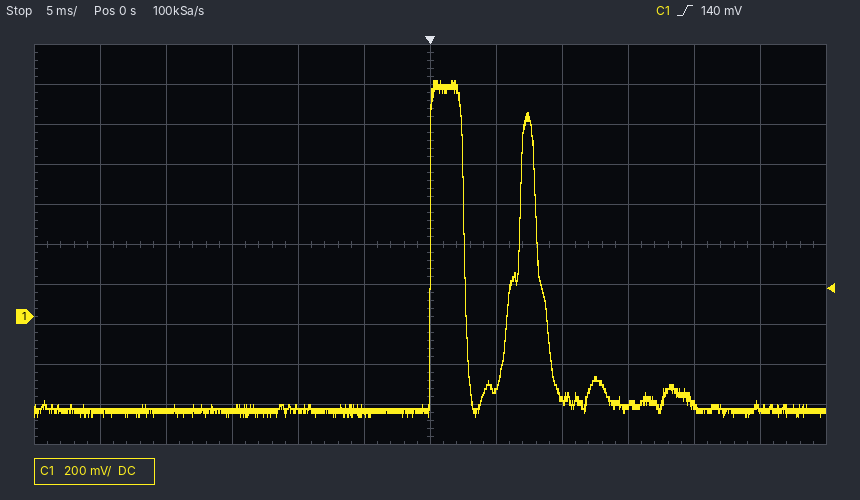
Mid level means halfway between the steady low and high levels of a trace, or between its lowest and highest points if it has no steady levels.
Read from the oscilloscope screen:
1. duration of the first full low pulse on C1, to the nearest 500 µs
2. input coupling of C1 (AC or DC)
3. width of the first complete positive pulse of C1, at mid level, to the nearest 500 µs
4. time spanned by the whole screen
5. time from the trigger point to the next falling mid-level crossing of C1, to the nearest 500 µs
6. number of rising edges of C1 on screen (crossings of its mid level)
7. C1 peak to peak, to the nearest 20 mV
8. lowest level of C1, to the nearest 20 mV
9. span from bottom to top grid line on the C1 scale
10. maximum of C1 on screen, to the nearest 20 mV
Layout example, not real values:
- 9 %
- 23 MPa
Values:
- 4.0 ms
- DC
- 2.5 ms
- 60 ms
- 2.5 ms
- 2
- 1.68 V
- -500 mV
- 2 V
- 1.18 V
